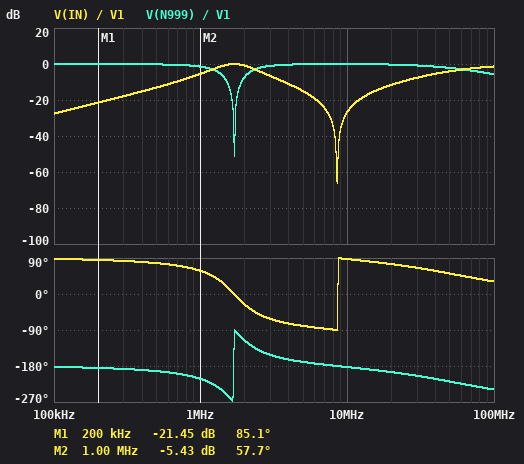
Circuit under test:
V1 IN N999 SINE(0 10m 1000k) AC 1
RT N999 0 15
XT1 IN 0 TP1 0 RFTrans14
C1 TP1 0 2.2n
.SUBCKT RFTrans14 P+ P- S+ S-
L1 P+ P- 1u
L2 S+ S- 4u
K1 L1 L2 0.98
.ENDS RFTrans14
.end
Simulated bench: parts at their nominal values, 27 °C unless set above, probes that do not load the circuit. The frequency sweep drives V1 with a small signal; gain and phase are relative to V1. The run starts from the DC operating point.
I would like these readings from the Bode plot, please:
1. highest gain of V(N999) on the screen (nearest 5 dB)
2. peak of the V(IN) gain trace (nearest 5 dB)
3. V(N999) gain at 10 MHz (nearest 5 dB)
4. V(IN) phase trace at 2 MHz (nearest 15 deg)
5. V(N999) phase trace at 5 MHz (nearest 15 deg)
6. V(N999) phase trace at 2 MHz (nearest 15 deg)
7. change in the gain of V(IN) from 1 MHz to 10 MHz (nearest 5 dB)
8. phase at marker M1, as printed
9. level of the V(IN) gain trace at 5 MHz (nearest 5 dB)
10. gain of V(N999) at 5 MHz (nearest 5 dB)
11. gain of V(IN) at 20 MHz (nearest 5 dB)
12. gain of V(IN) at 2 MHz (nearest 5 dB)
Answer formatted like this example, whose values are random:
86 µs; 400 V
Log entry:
0 dB; 0 dB; 0 dB; -30 deg; -165 deg; -120 deg; -20 dB; 85.1 deg; -15 dB; 0 dB; -10 dB; 0 dB
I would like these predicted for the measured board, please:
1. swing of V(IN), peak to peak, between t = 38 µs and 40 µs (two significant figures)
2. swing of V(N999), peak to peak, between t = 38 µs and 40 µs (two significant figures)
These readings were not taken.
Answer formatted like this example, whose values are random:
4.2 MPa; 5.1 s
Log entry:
11 mV; 17 mV
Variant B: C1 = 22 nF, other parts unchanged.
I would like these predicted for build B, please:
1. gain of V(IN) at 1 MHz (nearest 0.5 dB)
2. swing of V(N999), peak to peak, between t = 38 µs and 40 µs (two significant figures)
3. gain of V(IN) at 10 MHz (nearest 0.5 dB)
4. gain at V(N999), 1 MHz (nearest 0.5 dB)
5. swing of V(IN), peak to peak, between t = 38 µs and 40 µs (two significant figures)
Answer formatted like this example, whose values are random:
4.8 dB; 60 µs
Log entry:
-17.0 dB; 20 mV; -16.5 dB; 0 dB; 2.9 mV
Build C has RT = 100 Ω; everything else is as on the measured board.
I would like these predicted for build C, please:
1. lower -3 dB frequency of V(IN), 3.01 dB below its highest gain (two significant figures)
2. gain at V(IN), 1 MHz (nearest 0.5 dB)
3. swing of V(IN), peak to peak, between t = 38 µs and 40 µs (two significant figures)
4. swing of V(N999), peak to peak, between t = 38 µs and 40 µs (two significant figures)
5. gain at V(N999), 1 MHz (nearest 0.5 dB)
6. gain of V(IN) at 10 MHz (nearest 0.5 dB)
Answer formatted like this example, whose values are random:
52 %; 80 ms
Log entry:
1.6 MHz; -20.5 dB; 1.9 mV; 20 mV; 0 dB; -43.0 dB
